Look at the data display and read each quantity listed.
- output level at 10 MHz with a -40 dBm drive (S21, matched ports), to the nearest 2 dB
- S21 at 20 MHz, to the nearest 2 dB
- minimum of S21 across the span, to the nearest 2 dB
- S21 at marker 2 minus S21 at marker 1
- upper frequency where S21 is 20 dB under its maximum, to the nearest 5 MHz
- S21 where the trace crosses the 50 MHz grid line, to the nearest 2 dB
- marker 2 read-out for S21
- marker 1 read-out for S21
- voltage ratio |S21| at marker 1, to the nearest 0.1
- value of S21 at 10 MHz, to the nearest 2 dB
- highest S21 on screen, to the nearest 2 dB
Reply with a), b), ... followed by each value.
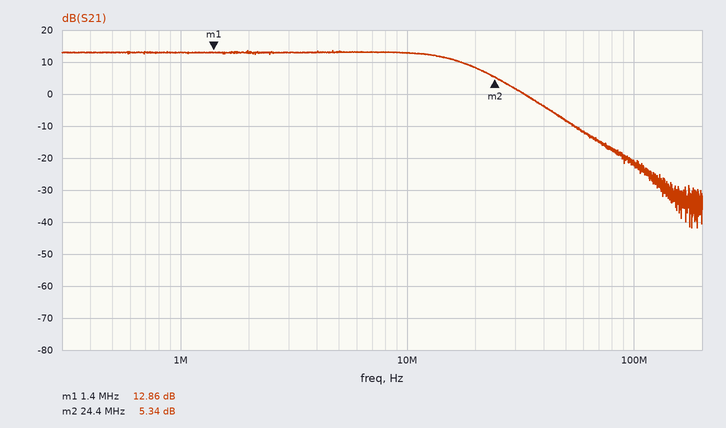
a) -28 dBm
b) 8 dB
c) -42 dB
d) -7.52 dB
e) 45 MHz
f) -8 dB
g) 5.34 dB
h) 12.86 dB
i) 4.4
j) 12 dB
k) 14 dB
